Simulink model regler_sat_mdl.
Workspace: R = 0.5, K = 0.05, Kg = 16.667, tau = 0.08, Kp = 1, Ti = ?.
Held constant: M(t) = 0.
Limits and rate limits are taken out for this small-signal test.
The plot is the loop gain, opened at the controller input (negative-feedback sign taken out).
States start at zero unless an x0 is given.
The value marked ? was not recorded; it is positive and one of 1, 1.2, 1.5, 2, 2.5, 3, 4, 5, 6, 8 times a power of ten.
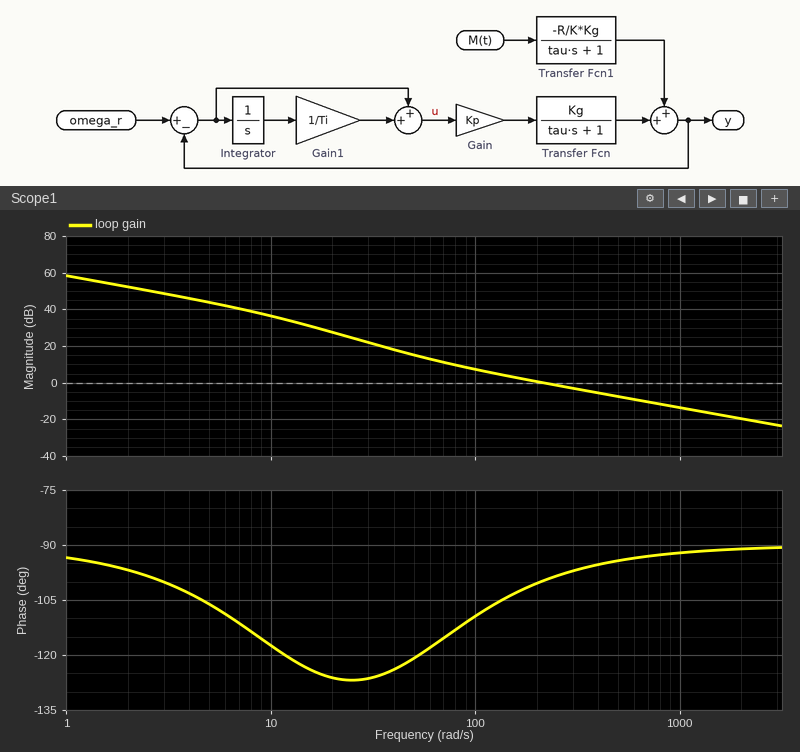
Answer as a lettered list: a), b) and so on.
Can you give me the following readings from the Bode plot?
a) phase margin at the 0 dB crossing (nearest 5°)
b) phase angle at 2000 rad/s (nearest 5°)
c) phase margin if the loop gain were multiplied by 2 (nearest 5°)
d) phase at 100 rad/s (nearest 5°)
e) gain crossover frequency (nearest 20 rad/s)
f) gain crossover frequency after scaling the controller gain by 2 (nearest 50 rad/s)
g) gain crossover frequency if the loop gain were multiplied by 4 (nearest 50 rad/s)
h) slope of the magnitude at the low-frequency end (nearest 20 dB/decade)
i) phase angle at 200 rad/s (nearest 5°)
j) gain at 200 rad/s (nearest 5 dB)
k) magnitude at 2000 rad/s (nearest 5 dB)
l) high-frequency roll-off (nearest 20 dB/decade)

a) 80°
b) -90°
c) 85°
d) -110°
e) 220 rad/s
f) 400 rad/s
g) 850 rad/s
h) -20 dB/decade
i) -100°
j) 0 dB
k) -20 dB
l) -20 dB/decade
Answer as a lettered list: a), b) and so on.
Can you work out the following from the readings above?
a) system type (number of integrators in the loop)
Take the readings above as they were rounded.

a) 1
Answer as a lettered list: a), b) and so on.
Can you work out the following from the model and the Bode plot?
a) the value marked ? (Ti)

a) 0.02
